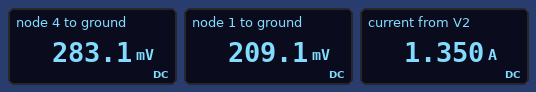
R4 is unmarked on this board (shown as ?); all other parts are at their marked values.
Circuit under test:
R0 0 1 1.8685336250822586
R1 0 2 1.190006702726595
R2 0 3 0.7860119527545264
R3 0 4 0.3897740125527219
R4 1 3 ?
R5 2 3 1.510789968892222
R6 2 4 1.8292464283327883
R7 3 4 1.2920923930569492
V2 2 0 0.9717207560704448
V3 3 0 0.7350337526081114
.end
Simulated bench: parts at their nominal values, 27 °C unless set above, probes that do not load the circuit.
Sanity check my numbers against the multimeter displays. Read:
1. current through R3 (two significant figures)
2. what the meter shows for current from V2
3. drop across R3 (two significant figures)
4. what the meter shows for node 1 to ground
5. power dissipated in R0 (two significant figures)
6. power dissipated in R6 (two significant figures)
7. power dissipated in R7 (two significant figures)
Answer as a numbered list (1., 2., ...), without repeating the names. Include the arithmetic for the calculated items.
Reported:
1. (283.1 mV) / 389.8 mΩ = 730 mA
2. 1.350 A
3. 283.1 mV = 280 mV
4. 209.1 mV
5. (209.1 mV)^2 / 1.869 Ω = 23 mW
6. (971.7 mV - 283.1 mV)^2 / 1.829 Ω = 260 mW
7. (735 mV - 283.1 mV)^2 / 1.292 Ω = 160 mW
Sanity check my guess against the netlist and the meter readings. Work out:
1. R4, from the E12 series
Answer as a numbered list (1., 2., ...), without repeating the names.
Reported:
1. 4.7 Ω
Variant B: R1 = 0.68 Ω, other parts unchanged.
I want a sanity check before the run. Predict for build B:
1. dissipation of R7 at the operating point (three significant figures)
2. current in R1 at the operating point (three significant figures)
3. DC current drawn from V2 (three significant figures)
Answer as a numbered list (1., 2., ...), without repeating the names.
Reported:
1. 158 mW
2. 1.43 A
3. 1.96 A
